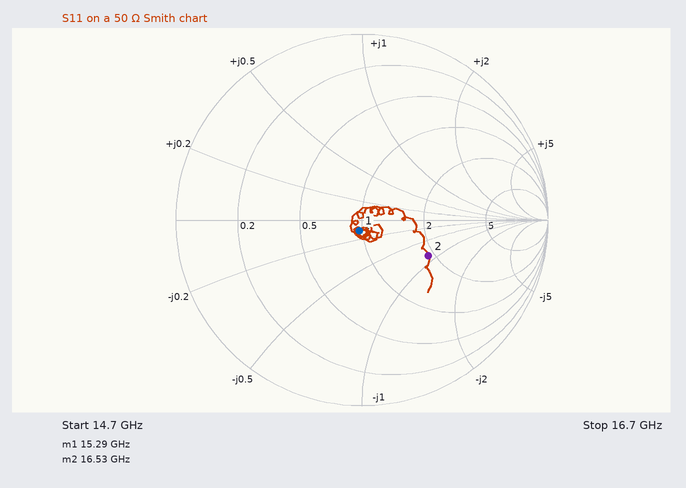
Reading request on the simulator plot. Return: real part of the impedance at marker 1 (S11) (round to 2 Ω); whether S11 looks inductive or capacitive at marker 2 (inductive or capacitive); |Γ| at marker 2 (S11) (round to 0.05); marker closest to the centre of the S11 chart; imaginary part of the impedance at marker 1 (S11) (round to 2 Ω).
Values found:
48 Ω
capacitive
0.40
marker 1
-6 Ω
